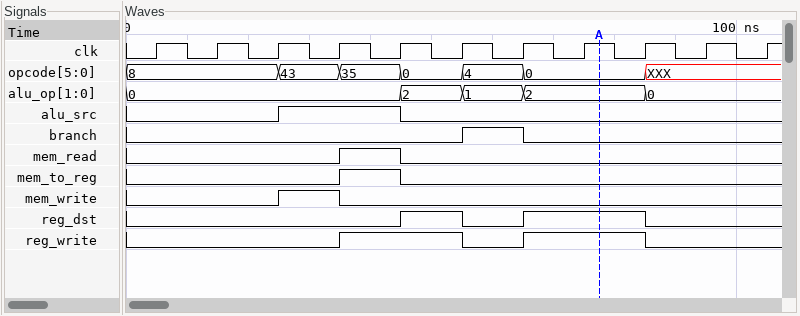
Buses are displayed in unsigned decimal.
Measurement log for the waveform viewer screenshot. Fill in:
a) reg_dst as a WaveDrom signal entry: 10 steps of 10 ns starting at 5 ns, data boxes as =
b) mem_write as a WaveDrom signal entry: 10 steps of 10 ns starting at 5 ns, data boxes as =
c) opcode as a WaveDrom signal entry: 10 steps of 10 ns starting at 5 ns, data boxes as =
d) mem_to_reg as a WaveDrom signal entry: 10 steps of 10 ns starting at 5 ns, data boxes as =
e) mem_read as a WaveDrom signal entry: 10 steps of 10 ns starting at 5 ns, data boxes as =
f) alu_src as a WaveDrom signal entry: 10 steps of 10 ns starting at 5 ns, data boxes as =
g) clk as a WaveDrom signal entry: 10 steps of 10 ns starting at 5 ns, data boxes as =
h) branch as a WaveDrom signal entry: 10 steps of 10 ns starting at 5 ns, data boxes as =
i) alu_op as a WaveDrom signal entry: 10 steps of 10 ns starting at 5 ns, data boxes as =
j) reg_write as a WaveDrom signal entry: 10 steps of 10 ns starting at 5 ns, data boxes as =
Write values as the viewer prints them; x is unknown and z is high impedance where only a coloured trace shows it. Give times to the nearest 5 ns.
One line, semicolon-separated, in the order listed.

{name: 'reg_dst', wave: '0...101.0.'}; {name: 'mem_write', wave: '0.10......'}; {name: 'opcode', wave: '=.=====.x.', data: '8 43 35 0 4 0'}; {name: 'mem_to_reg', wave: '0..10.....'}; {name: 'mem_read', wave: '0..10.....'}; {name: 'alu_src', wave: '0.1.0.....'}; {name: 'clk', wave: 'p.........'}; {name: 'branch', wave: '0....10...'}; {name: 'alu_op', wave: '=...===.=.', data: '0 2 1 2 0'}; {name: 'reg_write', wave: '0..1.01.0.'}
